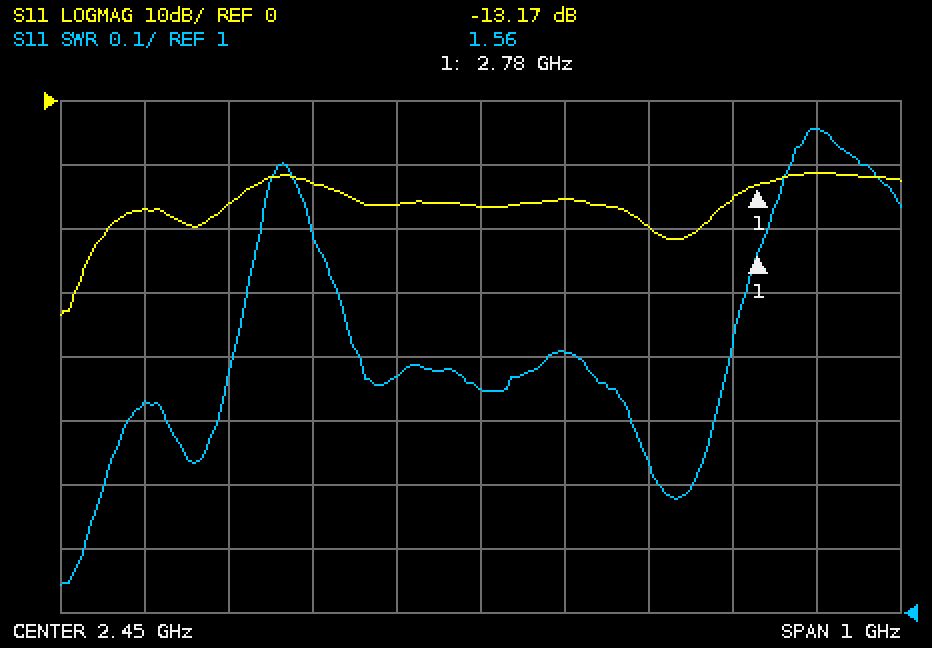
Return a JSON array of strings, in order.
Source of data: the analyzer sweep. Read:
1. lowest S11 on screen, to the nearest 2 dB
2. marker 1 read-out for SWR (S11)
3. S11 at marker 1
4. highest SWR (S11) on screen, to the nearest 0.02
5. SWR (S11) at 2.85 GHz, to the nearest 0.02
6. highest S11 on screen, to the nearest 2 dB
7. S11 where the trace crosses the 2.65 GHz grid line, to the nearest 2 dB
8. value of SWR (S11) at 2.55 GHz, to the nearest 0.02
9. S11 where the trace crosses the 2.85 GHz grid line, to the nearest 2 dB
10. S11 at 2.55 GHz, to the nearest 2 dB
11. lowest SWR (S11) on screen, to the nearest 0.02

["-34 dB", "1.56", "-13.17 dB", "1.76", "1.76", "-12 dB", "-20 dB", "1.40", "-12 dB", "-16 dB", "1.04"]
